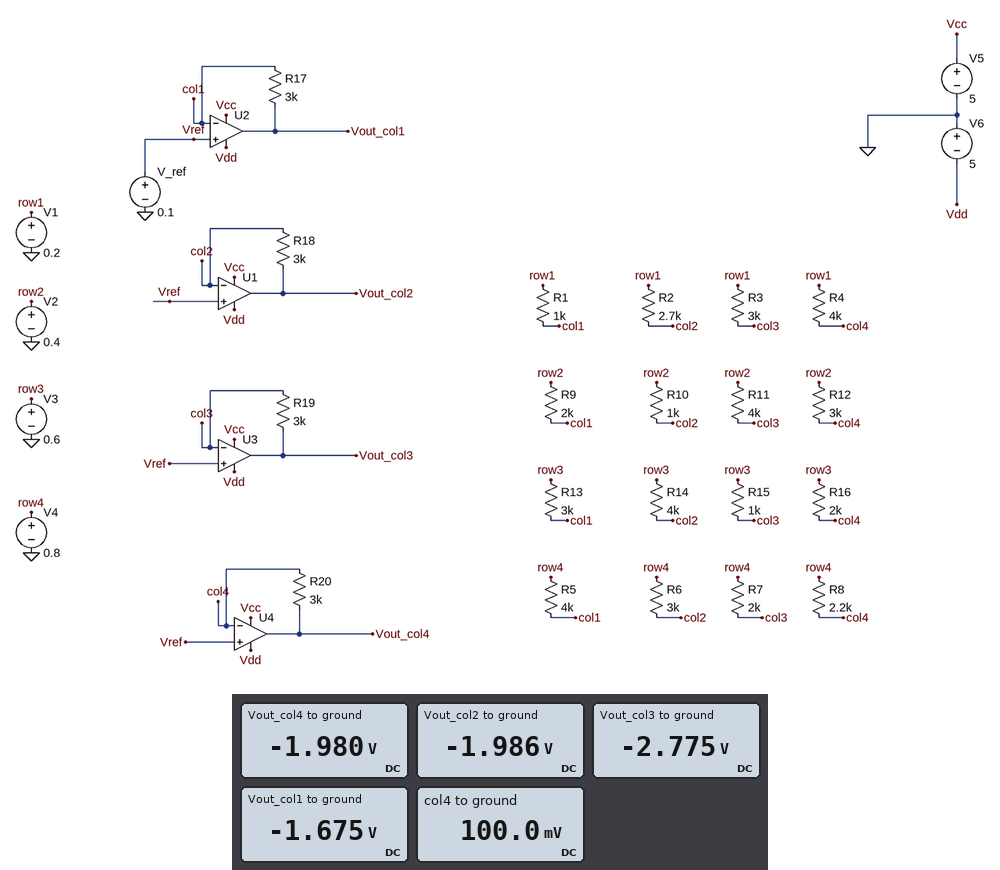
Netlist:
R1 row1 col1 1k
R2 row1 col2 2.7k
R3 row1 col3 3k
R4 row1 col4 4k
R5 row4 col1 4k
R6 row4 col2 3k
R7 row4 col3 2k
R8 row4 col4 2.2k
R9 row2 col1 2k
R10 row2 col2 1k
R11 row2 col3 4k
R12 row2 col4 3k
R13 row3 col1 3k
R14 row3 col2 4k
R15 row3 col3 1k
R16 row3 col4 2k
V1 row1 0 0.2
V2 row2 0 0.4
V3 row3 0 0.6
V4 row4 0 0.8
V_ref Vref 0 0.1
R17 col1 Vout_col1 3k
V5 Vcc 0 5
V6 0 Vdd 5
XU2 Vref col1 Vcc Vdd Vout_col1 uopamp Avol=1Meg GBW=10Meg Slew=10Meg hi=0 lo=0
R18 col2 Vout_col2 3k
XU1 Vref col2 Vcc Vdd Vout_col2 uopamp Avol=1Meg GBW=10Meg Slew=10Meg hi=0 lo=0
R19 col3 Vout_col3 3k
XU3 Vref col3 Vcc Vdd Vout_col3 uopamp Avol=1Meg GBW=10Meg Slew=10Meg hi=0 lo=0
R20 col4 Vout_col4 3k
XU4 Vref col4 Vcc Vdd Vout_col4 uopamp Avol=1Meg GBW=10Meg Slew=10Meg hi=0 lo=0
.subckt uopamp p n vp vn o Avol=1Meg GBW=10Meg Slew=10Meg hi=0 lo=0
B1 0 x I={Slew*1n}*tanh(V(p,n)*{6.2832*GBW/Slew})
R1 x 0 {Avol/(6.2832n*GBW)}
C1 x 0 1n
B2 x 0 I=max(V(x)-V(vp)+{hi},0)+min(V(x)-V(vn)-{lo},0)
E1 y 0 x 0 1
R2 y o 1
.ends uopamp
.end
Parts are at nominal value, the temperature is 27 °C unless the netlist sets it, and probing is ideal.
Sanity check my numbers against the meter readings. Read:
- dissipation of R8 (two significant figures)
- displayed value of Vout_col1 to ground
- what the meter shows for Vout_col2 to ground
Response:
220 µW
-1.675 V
-1.986 V
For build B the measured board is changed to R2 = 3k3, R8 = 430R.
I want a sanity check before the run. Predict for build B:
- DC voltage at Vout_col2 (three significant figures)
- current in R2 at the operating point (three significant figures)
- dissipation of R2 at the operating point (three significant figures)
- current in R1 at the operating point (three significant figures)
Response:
-1.97 V
30.3 µA
3.03 µW
100 µA
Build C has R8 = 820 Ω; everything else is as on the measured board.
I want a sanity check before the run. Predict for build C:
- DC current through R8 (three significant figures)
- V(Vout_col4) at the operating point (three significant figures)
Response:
854 µA
-3.59 V
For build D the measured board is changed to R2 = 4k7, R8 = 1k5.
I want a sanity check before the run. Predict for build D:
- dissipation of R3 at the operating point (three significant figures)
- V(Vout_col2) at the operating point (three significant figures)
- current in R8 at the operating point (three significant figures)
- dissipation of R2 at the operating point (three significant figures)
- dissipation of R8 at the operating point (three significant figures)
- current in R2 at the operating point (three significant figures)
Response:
3.33 µW
-1.94 V
467 µA
2.13 µW
327 µW
21.3 µA
